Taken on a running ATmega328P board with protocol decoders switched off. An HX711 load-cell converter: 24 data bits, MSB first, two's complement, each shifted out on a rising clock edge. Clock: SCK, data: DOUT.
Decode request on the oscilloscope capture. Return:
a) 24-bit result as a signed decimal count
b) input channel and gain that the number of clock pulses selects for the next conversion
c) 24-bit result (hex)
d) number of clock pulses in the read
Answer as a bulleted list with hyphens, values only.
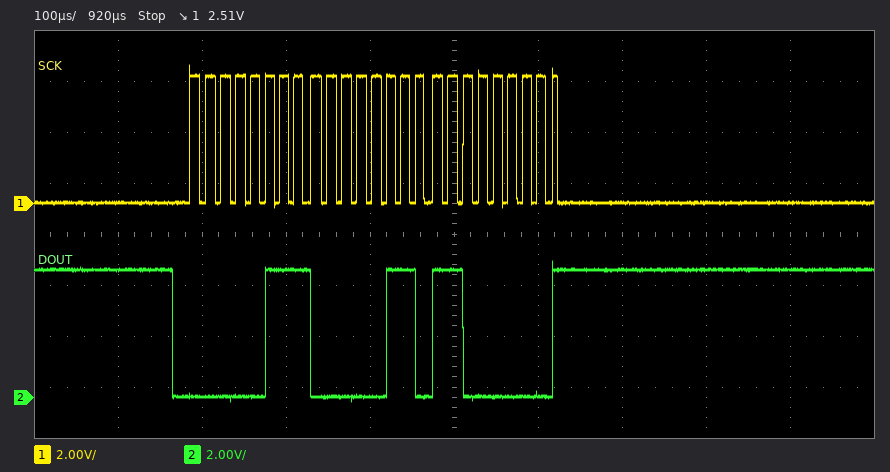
- 460480
- channel A, gain 128
- 0x0706C0
- 25
